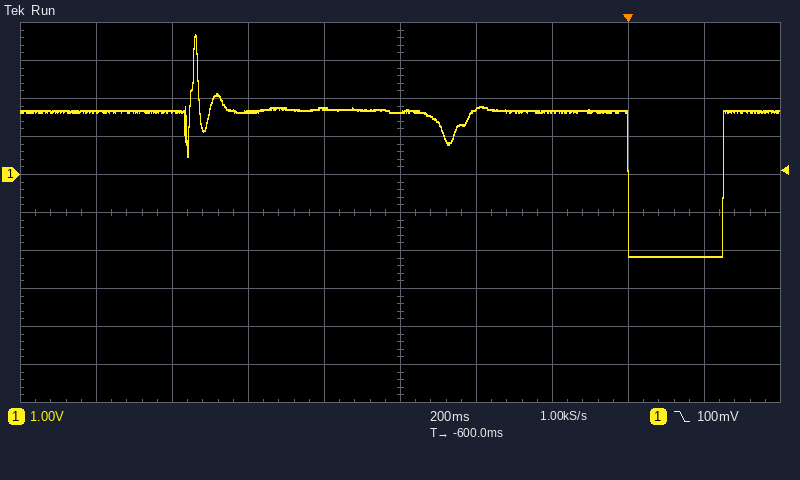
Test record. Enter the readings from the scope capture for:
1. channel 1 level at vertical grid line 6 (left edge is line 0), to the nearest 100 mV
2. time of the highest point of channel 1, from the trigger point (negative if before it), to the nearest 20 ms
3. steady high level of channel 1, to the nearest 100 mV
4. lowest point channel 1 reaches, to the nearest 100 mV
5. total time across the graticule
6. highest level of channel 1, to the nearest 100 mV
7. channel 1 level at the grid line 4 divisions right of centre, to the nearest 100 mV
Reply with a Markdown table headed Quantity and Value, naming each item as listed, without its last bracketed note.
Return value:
| Quantity | Value |
|---|---|
| channel 1 level at vertical grid line 6 (left edge is line 0), to the nearest 100 mV | 1.7 V |
| time of the highest point of channel 1, from the trigger point (negative if before it), to the nearest 20 ms | -1.14 s |
| steady high level of channel 1, to the nearest 100 mV | 1.7 V |
| lowest point channel 1 reaches, to the nearest 100 mV | -2.2 V |
| total time across the graticule | 2 s |
| highest level of channel 1, to the nearest 100 mV | 3.7 V |
| channel 1 level at the grid line 4 divisions right of centre, to the nearest 100 mV | -2.2 V |
